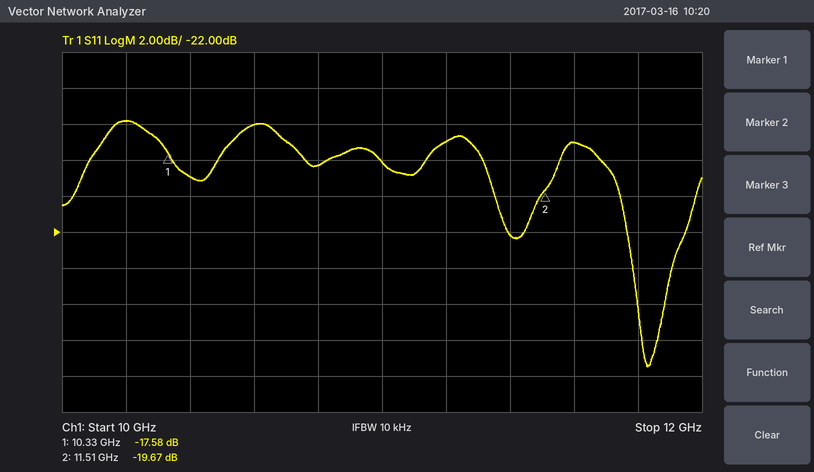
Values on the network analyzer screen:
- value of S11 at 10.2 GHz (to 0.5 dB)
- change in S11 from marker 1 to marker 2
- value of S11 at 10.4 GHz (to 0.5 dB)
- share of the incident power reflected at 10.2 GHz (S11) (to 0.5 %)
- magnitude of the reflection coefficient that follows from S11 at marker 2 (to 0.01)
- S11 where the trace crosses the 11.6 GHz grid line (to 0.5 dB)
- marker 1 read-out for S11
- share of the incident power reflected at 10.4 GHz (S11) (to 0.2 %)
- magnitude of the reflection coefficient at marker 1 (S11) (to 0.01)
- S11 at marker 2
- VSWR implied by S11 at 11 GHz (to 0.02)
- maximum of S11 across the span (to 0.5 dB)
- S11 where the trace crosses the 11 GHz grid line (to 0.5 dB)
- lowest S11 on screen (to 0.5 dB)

-16.0 dB
-2.09 dB
-19.0 dB
2.5 %
0.10
-17.0 dB
-17.58 dB
1.2 %
0.13
-19.67 dB
1.28
-16.0 dB
-18.0 dB
-29.5 dB
